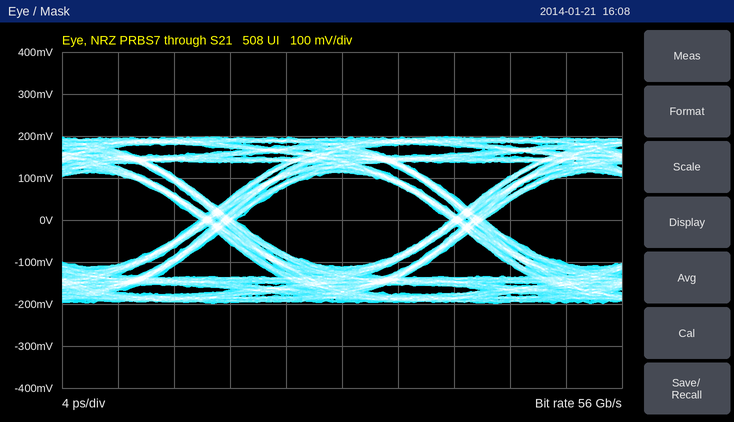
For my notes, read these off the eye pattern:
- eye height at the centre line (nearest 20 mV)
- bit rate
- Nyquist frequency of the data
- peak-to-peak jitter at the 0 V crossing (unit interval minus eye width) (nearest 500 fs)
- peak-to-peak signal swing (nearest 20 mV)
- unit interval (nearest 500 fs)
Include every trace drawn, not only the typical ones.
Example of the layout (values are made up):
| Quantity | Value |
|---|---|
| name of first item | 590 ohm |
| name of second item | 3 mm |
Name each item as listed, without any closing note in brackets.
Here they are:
| Quantity | Value |
|---|---|
| eye height at the centre line | 220 mV |
| bit rate | 56 Gb/s |
| Nyquist frequency of the data | 28 GHz |
| peak-to-peak jitter at the 0 V crossing (unit interval minus eye width) | 2.5 ps |
| peak-to-peak signal swing | 400 mV |
| unit interval | 18.0 ps |
